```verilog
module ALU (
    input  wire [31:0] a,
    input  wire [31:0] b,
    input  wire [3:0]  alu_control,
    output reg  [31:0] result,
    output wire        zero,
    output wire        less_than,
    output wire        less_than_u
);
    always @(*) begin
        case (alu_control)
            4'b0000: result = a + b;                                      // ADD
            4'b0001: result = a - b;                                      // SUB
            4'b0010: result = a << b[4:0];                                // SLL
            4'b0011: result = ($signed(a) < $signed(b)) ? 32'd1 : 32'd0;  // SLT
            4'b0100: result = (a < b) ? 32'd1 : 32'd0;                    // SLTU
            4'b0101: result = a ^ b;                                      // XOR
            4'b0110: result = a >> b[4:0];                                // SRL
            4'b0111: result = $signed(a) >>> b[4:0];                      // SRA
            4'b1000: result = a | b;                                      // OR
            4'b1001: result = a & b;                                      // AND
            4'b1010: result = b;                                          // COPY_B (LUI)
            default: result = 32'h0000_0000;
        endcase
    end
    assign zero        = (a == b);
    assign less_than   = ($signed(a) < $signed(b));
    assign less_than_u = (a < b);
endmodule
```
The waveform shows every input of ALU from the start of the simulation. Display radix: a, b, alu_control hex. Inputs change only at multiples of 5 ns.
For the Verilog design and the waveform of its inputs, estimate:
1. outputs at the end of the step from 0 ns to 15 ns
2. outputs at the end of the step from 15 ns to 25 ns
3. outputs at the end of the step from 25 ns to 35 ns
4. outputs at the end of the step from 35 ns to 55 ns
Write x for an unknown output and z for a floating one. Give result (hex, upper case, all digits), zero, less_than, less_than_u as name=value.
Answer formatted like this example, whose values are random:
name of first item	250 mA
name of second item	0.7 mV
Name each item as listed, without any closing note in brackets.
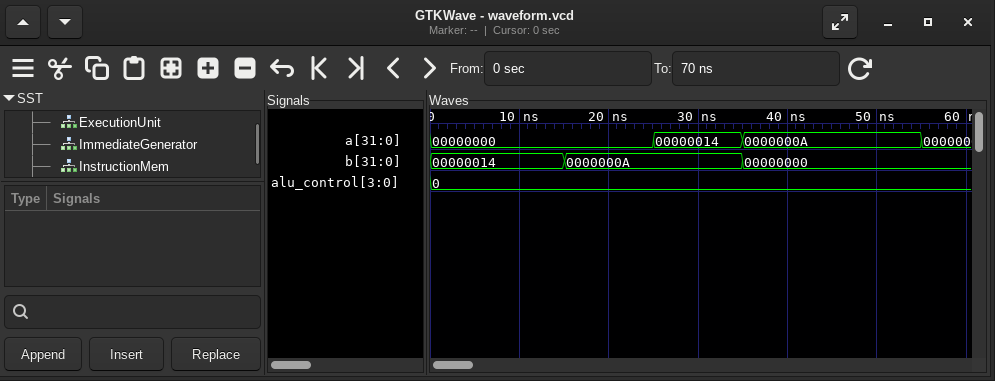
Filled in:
outputs at the end of the step from 0 ns to 15 ns	result=00000014, zero=0, less_than=1, less_than_u=1
outputs at the end of the step from 15 ns to 25 ns	result=0000000A, zero=0, less_than=1, less_than_u=1
outputs at the end of the step from 25 ns to 35 ns	result=0000001E, zero=0, less_than=0, less_than_u=0
outputs at the end of the step from 35 ns to 55 ns	result=0000000A, zero=0, less_than=0, less_than_u=0
